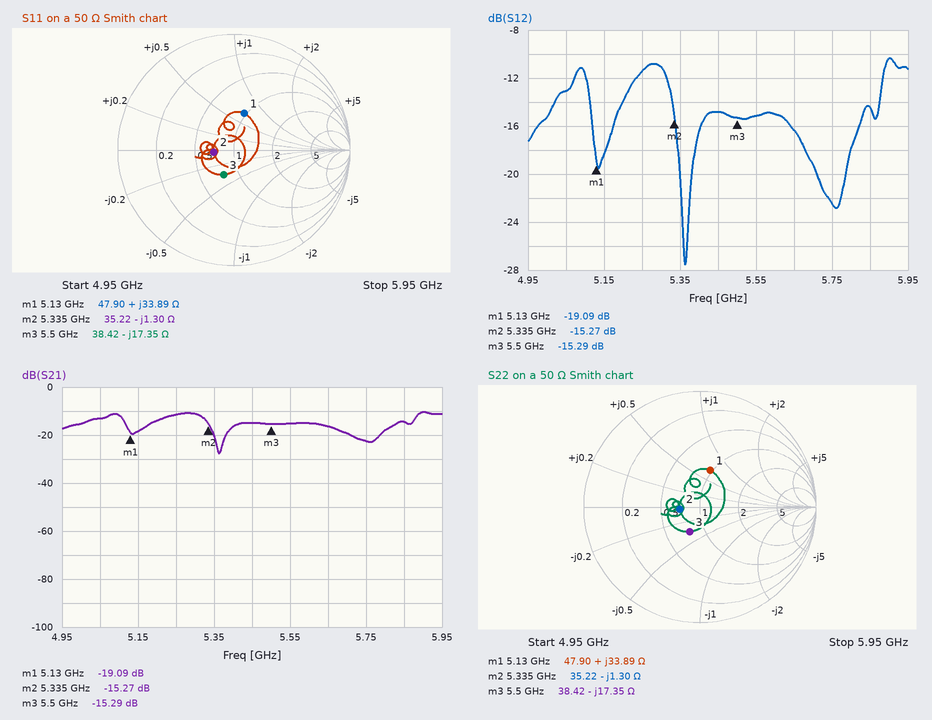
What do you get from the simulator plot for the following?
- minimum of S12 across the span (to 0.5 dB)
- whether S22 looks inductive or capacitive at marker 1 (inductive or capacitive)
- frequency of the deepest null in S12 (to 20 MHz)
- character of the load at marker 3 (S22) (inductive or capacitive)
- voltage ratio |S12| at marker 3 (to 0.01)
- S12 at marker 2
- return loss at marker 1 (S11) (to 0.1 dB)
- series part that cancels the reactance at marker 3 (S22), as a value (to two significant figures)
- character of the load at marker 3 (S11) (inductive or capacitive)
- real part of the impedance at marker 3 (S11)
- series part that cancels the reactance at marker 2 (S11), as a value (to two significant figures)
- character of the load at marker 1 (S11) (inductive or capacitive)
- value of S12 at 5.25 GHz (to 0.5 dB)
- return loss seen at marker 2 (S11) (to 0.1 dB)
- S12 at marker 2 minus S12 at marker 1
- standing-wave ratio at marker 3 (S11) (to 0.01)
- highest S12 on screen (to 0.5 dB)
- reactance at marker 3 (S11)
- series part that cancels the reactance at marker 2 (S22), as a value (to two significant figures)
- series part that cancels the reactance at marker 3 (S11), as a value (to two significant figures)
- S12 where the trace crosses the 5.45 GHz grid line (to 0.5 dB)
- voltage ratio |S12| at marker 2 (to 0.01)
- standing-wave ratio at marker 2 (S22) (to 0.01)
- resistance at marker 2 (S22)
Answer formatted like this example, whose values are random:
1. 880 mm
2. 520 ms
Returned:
1. -27.5 dB
2. inductive
3. 5.36 GHz
4. capacitive
5. 0.17
6. -15.27 dB
7. 9.7 dB
8. 500 pH
9. capacitive
10. 38.42 Ω
11. 39 pH
12. inductive
13. -11.5 dB
14. 15.2 dB
15. 3.82 dB
16. 1.60
17. -10.5 dB
18. -17.35 Ω
19. 39 pH
20. 500 pH
21. -15.0 dB
22. 0.17
23. 1.42
24. 35.22 Ω
